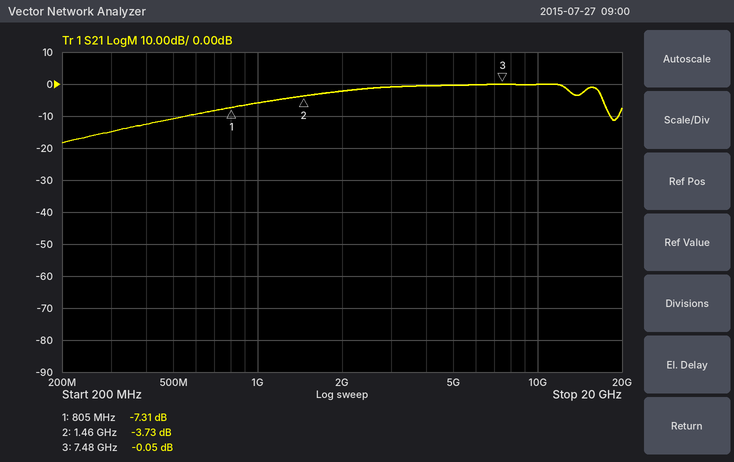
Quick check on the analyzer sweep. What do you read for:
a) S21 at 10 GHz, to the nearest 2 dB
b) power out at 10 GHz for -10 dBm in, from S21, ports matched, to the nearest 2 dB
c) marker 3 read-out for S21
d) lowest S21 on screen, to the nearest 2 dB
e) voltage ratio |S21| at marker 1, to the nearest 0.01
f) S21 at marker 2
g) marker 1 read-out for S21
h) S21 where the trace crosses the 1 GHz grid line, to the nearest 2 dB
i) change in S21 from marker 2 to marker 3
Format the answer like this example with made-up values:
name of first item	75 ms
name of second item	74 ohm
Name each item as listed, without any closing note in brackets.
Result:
S21 at 10 GHz, to the nearest 2 dB	0 dB
power out at 10 GHz for -10 dBm in, from S21, ports matched, to the nearest 2 dB	-10 dBm
marker 3 read-out for S21	-0.05 dB
lowest S21 on screen, to the nearest 2 dB	-18 dB
voltage ratio |S21| at marker 1, to the nearest 0.01	0.43
S21 at marker 2	-3.73 dB
marker 1 read-out for S21	-7.31 dB
S21 where the trace crosses the 1 GHz grid line, to the nearest 2 dB	-6 dB
change in S21 from marker 2 to marker 3	3.68 dB
